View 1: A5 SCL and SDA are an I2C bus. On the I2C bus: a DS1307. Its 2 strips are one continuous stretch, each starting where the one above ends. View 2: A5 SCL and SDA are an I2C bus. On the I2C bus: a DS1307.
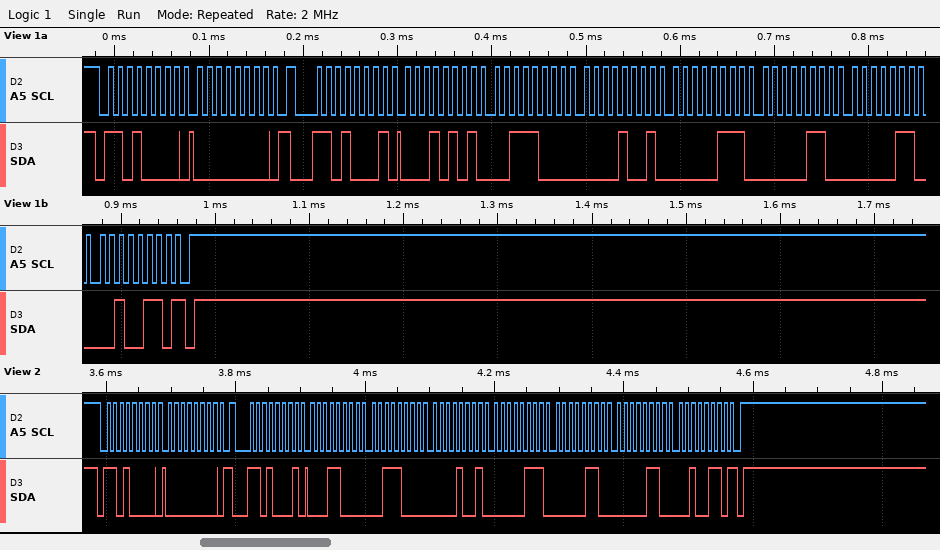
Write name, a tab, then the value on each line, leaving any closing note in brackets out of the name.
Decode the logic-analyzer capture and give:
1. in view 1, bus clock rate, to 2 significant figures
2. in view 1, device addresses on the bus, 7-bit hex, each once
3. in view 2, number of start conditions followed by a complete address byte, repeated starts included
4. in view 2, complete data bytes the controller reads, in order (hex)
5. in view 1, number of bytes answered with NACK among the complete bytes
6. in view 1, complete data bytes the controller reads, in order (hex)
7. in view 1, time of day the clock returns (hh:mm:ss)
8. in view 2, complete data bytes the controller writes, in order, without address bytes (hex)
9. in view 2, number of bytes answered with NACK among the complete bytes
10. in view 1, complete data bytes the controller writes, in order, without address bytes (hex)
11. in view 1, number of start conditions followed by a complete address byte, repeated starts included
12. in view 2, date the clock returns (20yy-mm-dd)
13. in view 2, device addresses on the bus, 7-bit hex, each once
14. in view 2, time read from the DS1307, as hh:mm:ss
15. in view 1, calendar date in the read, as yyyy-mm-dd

in view 1, bus clock rate, to 2 significant figures	100 kHz
in view 1, device addresses on the bus, 7-bit hex, each once	0x68
in view 2, number of start conditions followed by a complete address byte, repeated starts included	2
in view 2, complete data bytes the controller reads, in order	18 38 09 07 06 06 26
in view 1, number of bytes answered with NACK among the complete bytes	1
in view 1, complete data bytes the controller reads, in order	15 38 09 07 06 06 26
in view 1, time of day the clock returns	09:38:15
in view 2, complete data bytes the controller writes, in order, without address bytes	00
in view 2, number of bytes answered with NACK among the complete bytes	1
in view 1, complete data bytes the controller writes, in order, without address bytes	00
in view 1, number of start conditions followed by a complete address byte, repeated starts included	2
in view 2, date the clock returns	2026-06-06
in view 2, device addresses on the bus, 7-bit hex, each once	0x68
in view 2, time read from the DS1307, as hh:mm:ss	09:38:18
in view 1, calendar date in the read, as yyyy-mm-dd	2026-06-06
